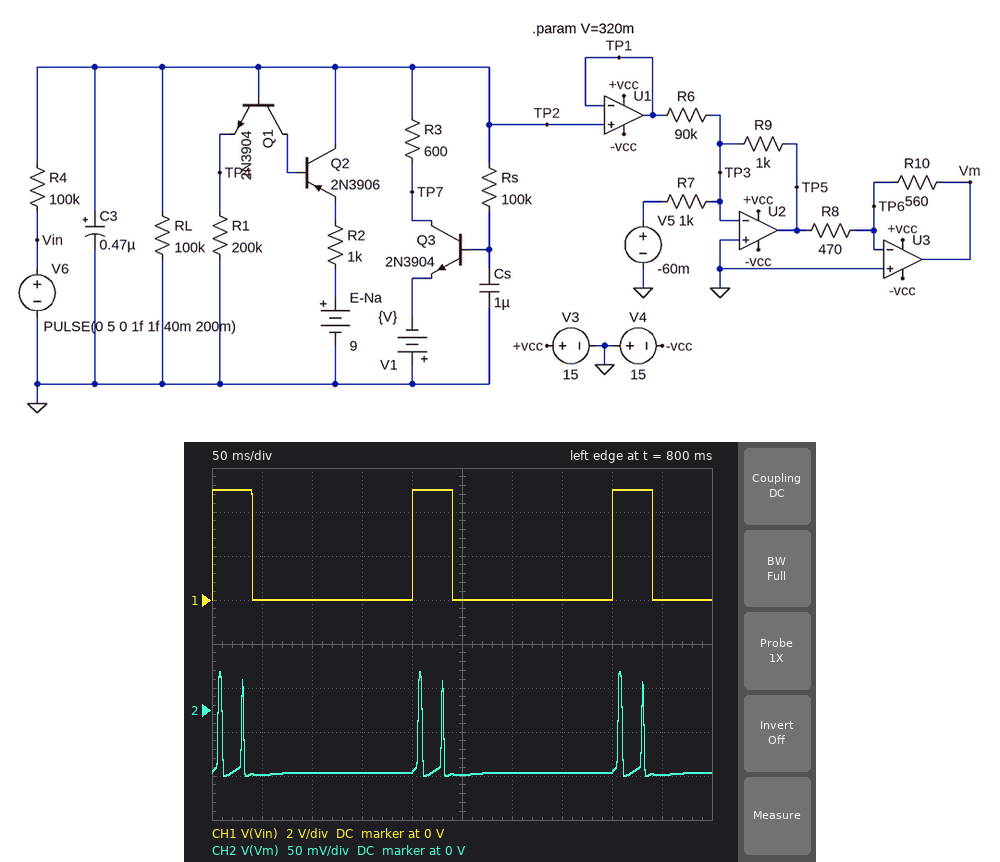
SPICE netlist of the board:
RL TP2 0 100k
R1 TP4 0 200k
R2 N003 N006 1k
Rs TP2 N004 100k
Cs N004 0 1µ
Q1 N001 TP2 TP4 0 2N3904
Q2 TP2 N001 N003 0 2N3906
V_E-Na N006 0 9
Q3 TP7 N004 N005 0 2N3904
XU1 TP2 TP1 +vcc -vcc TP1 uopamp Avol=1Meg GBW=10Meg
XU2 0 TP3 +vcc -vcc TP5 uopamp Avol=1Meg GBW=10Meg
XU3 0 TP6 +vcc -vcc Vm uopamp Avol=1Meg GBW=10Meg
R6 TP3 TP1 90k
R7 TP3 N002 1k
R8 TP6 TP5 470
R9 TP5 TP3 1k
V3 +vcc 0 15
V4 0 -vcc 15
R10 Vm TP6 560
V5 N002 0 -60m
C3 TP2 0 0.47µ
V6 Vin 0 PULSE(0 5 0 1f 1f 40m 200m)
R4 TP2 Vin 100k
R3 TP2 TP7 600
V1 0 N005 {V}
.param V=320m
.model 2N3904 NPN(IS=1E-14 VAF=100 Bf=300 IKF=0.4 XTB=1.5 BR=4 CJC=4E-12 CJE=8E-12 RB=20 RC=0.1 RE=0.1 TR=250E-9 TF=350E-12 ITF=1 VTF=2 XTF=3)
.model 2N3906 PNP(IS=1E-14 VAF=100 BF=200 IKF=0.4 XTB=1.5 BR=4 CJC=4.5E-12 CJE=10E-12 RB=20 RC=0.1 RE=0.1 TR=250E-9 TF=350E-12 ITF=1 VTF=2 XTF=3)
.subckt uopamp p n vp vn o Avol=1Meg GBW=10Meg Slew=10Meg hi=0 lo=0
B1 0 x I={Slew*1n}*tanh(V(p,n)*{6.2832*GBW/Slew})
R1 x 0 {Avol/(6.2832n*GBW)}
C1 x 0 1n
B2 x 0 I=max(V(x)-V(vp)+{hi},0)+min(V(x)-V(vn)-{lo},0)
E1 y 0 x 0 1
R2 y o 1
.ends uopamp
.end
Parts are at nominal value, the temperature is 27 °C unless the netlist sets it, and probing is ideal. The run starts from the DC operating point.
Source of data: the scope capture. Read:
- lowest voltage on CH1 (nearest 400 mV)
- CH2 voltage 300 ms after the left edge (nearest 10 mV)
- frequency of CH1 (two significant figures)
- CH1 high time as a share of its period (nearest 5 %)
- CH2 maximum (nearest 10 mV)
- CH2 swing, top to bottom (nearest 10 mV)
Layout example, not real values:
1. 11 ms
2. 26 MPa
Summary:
1. 0 V
2. -70 mV
3. 5.0 Hz
4. 20 %
5. 40 mV
6. 120 mV
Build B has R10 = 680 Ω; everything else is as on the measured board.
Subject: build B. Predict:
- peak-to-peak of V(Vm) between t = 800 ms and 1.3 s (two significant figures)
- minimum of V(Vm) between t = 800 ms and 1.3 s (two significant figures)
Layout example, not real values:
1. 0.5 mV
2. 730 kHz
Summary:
1. 140 mV
2. -91 mV
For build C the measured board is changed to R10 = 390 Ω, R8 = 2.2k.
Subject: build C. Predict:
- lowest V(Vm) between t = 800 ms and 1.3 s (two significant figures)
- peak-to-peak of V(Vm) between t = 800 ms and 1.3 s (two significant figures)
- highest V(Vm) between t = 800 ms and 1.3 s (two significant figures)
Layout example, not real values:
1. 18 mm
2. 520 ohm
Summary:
1. -11 mV
2. 18 mV
3. 6.4 mV
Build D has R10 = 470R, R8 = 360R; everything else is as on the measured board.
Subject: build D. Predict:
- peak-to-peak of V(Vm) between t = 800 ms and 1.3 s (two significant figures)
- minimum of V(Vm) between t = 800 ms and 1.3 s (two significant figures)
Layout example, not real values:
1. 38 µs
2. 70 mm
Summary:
1. 130 mV
2. -82 mV
